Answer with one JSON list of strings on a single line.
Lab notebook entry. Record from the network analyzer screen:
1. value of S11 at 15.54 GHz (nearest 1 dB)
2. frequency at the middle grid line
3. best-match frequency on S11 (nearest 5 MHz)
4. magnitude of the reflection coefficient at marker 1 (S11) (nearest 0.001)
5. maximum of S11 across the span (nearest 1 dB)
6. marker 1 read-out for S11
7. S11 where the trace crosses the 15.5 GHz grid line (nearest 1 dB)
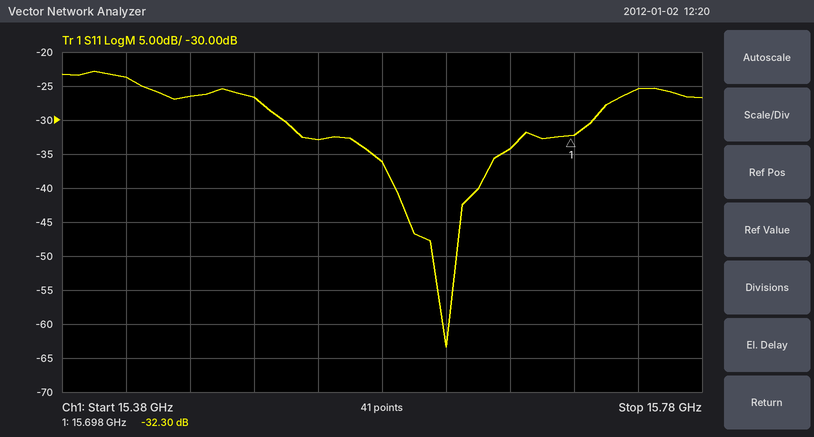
["-33 dB", "15.58 GHz", "15.620 GHz", "0.024", "-23 dB", "-32.30 dB", "-27 dB"]
